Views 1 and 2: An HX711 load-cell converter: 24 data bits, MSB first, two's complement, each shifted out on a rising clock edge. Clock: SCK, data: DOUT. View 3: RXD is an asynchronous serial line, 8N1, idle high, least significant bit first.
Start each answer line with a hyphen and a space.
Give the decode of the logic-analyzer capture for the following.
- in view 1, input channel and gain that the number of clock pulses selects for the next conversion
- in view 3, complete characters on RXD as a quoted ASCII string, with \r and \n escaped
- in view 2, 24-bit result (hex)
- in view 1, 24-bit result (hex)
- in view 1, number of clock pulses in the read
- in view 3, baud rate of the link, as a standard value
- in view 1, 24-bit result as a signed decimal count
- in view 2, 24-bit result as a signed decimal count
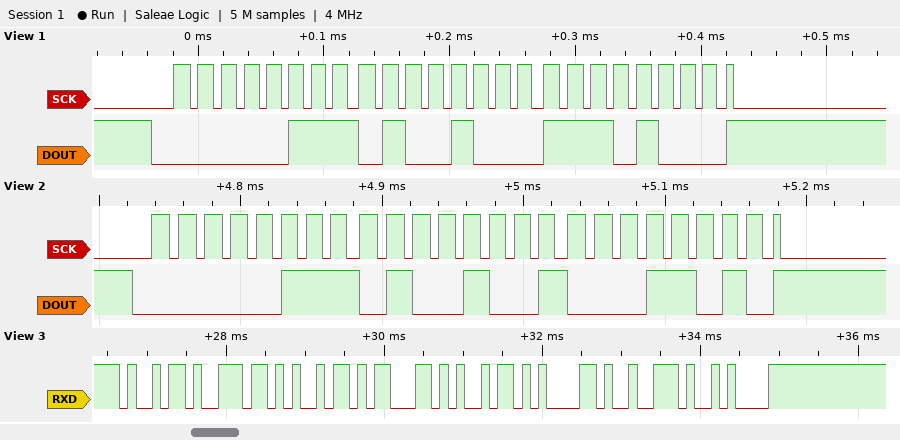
- channel A, gain 128
- "iniciar\n"
- 0x07491A
- 0x0748E8
- 25
- 9600 baud
- 477416
- 477466
